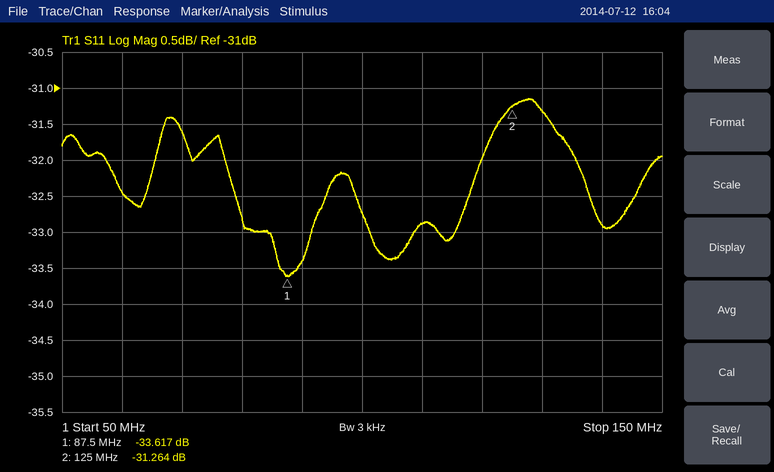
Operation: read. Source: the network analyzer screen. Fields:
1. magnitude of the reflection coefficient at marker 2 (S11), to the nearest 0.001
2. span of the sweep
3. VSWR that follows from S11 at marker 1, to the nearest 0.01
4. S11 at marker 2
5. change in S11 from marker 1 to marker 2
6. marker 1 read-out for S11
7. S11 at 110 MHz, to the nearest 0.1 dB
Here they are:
0.027
100 MHz
1.04
-31.264 dB
2.353 dB
-33.617 dB
-32.9 dB
